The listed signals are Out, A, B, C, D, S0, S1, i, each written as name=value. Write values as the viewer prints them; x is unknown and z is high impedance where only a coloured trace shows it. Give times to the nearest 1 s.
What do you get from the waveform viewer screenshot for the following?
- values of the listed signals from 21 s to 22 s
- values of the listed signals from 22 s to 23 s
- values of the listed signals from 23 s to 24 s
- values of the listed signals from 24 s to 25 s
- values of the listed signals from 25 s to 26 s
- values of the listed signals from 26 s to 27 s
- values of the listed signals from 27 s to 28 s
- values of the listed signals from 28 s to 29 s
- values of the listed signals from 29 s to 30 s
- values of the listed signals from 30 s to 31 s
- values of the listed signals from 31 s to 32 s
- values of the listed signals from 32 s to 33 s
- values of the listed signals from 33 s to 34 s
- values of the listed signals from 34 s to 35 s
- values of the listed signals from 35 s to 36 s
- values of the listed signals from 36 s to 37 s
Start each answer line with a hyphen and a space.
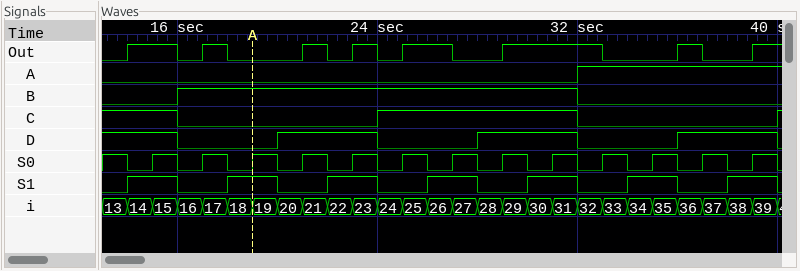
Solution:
- Out=1, A=0, B=1, C=0, D=1, S0=1, S1=0, i=21
- Out=0, A=0, B=1, C=0, D=1, S0=0, S1=1, i=22
- Out=1, A=0, B=1, C=0, D=1, S0=1, S1=1, i=23
- Out=0, A=0, B=1, C=1, D=0, S0=0, S1=0, i=24
- Out=1, A=0, B=1, C=1, D=0, S0=1, S1=0, i=25
- Out=1, A=0, B=1, C=1, D=0, S0=0, S1=1, i=26
- Out=0, A=0, B=1, C=1, D=0, S0=1, S1=1, i=27
- Out=0, A=0, B=1, C=1, D=1, S0=0, S1=0, i=28
- Out=1, A=0, B=1, C=1, D=1, S0=1, S1=0, i=29
- Out=1, A=0, B=1, C=1, D=1, S0=0, S1=1, i=30
- Out=1, A=0, B=1, C=1, D=1, S0=1, S1=1, i=31
- Out=1, A=1, B=0, C=0, D=0, S0=0, S1=0, i=32
- Out=0, A=1, B=0, C=0, D=0, S0=1, S1=0, i=33
- Out=0, A=1, B=0, C=0, D=0, S0=0, S1=1, i=34
- Out=0, A=1, B=0, C=0, D=0, S0=1, S1=1, i=35
- Out=1, A=1, B=0, C=0, D=1, S0=0, S1=0, i=36
